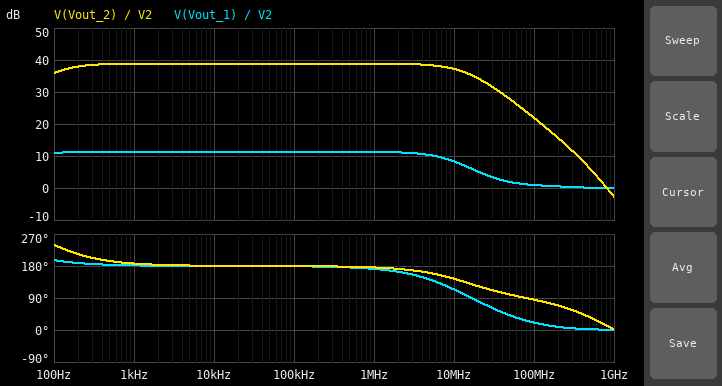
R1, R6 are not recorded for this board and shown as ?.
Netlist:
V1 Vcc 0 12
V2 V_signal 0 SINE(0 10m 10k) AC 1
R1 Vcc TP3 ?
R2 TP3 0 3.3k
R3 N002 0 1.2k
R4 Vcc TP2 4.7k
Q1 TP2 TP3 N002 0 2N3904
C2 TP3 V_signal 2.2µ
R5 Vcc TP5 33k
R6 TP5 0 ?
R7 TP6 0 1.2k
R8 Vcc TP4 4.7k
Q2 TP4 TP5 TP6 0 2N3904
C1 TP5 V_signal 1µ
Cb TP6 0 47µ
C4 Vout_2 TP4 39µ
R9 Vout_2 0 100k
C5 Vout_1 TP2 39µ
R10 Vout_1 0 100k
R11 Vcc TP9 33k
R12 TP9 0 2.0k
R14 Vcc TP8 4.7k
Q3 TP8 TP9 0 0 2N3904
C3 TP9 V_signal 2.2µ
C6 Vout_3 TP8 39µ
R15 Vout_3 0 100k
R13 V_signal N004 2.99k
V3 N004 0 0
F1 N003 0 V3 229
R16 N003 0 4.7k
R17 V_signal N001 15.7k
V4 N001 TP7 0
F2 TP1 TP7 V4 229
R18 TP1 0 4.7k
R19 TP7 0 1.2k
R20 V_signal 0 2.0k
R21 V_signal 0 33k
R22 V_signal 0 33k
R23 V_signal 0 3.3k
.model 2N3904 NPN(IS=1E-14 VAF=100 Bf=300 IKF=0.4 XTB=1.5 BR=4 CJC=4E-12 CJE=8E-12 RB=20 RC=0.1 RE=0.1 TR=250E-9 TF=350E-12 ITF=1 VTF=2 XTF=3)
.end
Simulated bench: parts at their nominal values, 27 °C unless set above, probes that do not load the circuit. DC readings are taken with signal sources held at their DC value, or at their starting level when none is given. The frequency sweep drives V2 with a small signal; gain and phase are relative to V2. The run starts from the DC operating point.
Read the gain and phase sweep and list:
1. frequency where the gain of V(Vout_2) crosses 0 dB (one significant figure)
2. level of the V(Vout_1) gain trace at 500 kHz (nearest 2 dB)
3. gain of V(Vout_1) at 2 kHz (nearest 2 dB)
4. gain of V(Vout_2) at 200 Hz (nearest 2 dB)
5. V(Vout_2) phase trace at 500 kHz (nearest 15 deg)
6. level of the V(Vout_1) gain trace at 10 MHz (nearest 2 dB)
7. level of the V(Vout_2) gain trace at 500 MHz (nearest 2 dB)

800 MHz
12 dB
12 dB
38 dB
180 deg
8 dB
6 dB
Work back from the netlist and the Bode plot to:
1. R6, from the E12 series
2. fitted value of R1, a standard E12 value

3.9 kΩ
10 kΩ
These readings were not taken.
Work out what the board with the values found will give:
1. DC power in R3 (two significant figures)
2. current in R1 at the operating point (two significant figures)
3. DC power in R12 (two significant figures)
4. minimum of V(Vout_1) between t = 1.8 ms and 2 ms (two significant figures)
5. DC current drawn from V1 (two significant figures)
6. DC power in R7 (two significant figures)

4.4 mW
900 µA
230 µW
-37 mV
6.0 mA
330 µW
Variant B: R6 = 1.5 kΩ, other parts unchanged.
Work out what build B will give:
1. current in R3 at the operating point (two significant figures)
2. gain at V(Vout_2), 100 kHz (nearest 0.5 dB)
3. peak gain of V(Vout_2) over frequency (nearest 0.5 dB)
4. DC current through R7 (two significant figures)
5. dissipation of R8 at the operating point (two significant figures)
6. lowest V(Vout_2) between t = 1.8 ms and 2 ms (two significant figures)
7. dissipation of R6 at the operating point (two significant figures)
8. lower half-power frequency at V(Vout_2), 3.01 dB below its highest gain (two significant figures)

1.9 mA
-1.0 dB
0 dB
5.1 µA
120 nW
-11 mV
180 µW
140 Hz
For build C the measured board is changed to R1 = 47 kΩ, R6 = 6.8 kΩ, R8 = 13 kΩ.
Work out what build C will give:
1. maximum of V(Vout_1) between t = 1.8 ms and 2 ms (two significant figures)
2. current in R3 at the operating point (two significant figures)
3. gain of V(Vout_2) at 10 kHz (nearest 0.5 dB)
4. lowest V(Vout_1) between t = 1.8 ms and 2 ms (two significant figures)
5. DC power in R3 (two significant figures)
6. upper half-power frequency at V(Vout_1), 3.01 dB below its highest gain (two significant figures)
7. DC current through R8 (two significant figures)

33 mV
150 µA
8.5 dB
-33 mV
28 µW
26 MHz
840 µA
